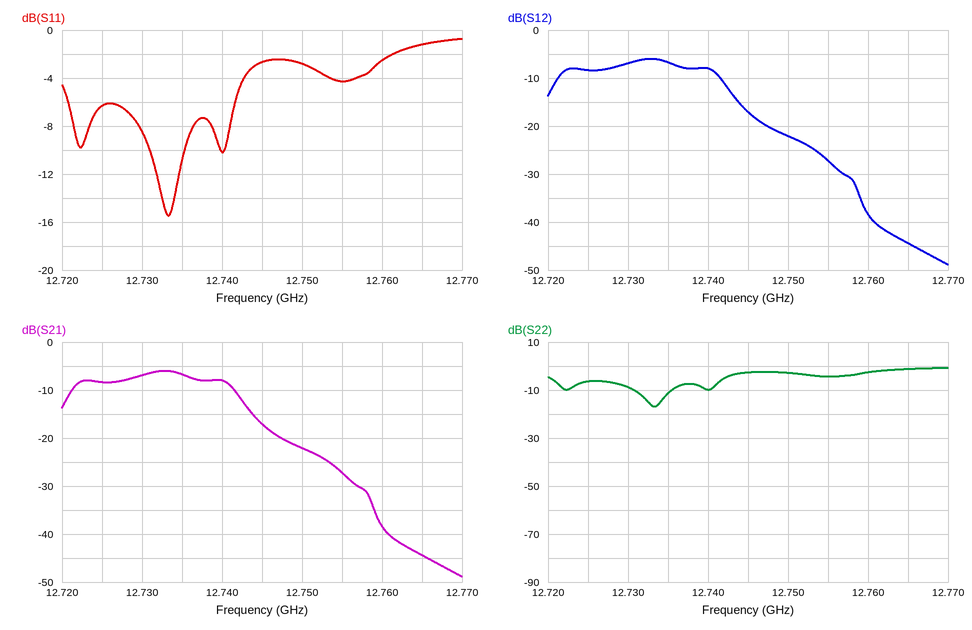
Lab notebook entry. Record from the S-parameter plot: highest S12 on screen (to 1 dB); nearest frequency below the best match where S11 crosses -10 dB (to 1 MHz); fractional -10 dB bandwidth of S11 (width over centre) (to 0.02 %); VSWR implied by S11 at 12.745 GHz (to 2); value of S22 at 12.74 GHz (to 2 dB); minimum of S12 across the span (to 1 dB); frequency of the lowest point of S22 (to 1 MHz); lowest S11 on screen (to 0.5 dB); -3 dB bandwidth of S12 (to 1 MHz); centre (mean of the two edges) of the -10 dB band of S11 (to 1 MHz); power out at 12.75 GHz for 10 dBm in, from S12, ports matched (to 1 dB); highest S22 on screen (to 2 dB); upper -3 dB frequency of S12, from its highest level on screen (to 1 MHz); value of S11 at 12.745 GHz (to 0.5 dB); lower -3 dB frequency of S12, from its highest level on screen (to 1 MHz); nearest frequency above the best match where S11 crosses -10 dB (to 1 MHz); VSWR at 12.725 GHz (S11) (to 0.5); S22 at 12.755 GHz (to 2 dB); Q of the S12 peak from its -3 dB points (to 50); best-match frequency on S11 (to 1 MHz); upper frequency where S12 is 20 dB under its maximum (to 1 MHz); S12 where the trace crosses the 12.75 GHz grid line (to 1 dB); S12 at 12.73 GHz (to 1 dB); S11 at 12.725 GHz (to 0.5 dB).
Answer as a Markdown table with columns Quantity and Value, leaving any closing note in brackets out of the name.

| Quantity | Value |
|---|---|
| highest S12 on screen | -6 dB |
| nearest frequency below the best match where S11 crosses -10 dB | 12.731 GHz |
| fractional -10 dB bandwidth of S11 (width over centre) | 0.04 % |
| VSWR implied by S11 at 12.745 GHz | 6 |
| value of S22 at 12.74 GHz | -10 dB |
| minimum of S12 across the span | -49 dB |
| frequency of the lowest point of S22 | 12.733 GHz |
| lowest S11 on screen | -15.5 dB |
| -3 dB bandwidth of S12 | 19 MHz |
| centre (mean of the two edges) of the -10 dB band of S11 | 12.733 GHz |
| power out at 12.75 GHz for 10 dBm in, from S12, ports matched | -12 dBm |
| highest S22 on screen | 0 dB |
| upper -3 dB frequency of S12, from its highest level on screen | 12.741 GHz |
| value of S11 at 12.745 GHz | -2.5 dB |
| lower -3 dB frequency of S12, from its highest level on screen | 12.722 GHz |
| nearest frequency above the best match where S11 crosses -10 dB | 12.735 GHz |
| VSWR at 12.725 GHz (S11) | 3.0 |
| S22 at 12.755 GHz | -4 dB |
| Q of the S12 peak from its -3 dB points | 650 |
| best-match frequency on S11 | 12.733 GHz |
| upper frequency where S12 is 20 dB under its maximum | 12.754 GHz |
| S12 where the trace crosses the 12.75 GHz grid line | -22 dB |
| S12 at 12.73 GHz | -7 dB |
| S11 at 12.725 GHz | -6.5 dB |
